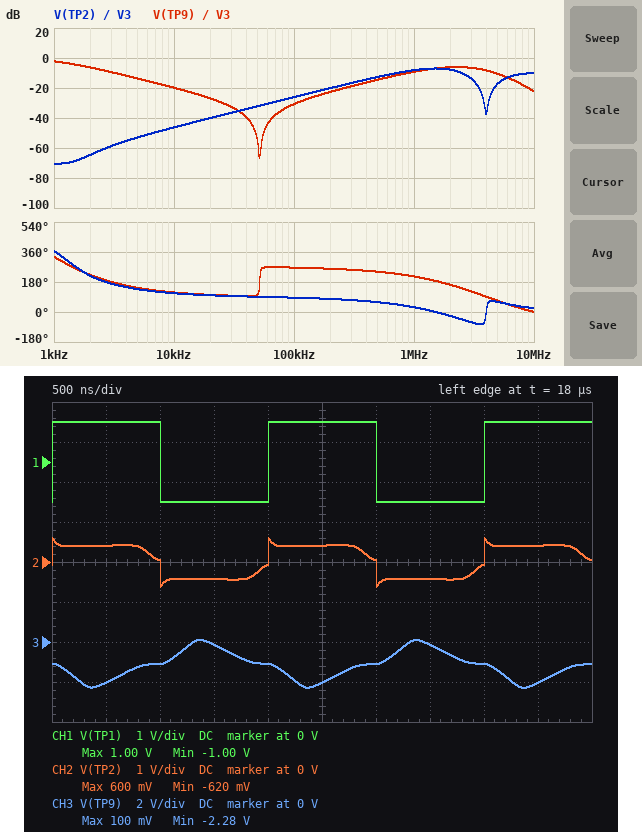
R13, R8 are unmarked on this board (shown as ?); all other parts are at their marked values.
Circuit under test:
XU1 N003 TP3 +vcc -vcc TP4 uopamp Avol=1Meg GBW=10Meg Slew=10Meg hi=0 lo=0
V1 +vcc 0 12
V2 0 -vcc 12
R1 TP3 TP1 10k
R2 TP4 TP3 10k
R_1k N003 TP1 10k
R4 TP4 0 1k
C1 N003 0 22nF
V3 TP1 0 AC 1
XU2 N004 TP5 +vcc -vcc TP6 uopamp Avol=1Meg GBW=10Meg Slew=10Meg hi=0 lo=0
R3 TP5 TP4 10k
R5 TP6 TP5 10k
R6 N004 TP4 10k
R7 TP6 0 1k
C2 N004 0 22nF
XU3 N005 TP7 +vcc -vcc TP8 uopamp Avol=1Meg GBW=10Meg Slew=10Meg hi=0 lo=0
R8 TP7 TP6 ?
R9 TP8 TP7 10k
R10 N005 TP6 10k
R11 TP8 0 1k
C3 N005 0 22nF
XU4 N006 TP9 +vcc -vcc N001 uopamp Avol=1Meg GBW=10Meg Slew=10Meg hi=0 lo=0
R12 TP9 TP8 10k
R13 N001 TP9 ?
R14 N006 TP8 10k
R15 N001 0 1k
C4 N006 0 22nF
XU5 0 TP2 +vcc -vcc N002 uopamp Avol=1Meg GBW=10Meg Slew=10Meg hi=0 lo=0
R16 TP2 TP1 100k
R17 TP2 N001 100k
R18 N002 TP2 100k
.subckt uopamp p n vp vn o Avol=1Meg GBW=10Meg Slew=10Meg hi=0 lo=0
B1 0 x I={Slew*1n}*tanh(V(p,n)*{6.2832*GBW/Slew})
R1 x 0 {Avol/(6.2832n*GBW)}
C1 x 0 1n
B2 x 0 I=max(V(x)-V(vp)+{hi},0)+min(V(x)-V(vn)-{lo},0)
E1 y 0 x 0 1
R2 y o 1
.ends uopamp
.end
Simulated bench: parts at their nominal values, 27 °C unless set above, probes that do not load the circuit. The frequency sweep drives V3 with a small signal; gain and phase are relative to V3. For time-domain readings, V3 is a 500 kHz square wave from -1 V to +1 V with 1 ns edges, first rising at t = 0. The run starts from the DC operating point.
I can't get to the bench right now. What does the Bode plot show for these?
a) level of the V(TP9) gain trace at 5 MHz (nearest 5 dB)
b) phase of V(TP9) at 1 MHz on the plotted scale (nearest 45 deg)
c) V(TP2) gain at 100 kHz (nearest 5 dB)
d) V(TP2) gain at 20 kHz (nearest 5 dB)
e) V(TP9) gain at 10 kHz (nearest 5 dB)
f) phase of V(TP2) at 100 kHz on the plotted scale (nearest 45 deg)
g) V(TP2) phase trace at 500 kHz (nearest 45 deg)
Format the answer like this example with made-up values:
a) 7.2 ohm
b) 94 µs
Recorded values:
a) -10 dB
b) 225 deg
c) -25 dB
d) -40 dB
e) -20 dB
f) 90 deg
g) 45 deg
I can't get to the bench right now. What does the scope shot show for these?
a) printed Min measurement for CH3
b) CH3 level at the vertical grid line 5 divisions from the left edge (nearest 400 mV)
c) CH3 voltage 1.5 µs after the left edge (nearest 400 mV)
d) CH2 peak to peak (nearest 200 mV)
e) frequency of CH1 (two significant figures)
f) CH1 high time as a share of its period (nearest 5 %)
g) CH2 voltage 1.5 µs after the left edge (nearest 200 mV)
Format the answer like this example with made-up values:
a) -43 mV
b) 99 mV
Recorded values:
a) -2.28 V
b) -2.0 V
c) 0 V
d) 1.2 V
e) 500 kHz
f) 50 %
g) -400 mV
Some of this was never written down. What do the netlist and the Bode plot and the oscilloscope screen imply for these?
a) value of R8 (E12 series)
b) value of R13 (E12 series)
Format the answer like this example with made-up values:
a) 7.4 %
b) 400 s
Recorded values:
a) 6.8 kΩ
b) 27 kΩ
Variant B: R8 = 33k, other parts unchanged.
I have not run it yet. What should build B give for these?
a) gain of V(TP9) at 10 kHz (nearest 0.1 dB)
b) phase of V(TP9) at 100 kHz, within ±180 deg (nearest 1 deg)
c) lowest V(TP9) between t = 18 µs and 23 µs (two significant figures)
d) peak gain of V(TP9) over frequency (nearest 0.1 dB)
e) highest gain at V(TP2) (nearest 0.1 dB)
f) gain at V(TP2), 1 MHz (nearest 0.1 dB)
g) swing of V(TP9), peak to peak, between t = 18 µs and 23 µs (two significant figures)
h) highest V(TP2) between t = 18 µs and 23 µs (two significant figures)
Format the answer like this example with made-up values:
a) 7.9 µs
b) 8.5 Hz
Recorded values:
a) -33.3 dB
b) -92 deg
c) -1.1 V
d) 0 dB
e) -9.5 dB
f) -16.4 dB
g) 230 mV
h) 660 mV
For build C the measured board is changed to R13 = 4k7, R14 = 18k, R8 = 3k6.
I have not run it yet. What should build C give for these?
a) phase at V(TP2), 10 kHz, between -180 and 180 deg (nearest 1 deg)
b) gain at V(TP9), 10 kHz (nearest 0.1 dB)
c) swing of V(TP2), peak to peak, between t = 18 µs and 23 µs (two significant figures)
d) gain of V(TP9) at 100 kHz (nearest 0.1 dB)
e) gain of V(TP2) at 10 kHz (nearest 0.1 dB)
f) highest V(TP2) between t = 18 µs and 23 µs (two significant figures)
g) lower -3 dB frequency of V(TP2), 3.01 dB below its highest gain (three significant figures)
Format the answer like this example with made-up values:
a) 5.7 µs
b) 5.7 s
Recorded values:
a) 106 deg
b) -19.2 dB
c) 1.3 V
d) -54.4 dB
e) -53.0 dB
f) 660 mV
g) 5.59 MHz
